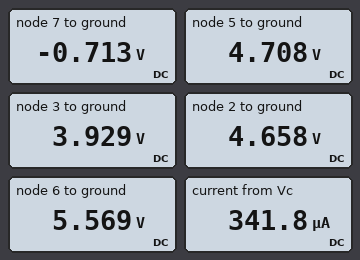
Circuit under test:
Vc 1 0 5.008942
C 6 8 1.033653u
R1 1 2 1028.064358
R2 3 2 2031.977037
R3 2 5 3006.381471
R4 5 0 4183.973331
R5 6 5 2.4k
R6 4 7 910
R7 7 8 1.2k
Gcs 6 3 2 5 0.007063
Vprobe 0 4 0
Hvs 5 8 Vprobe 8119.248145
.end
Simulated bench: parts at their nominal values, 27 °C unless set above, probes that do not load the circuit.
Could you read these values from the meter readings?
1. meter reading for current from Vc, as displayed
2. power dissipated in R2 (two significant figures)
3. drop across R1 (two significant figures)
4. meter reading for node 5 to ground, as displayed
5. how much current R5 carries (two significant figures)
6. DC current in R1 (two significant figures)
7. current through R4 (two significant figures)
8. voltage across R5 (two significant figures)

341.8 µA
260 µW
350 mV
4.708 V
360 µA
340 µA
1.1 mA
860 mV
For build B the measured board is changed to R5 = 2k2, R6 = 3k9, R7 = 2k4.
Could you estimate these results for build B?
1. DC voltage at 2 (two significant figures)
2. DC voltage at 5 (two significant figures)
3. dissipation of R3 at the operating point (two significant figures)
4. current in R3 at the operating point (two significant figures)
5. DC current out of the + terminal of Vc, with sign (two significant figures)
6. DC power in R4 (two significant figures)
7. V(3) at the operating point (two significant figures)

7.2 V
6.9 V
34 µW
110 µA
-2.1 mA
11 mW
12 V
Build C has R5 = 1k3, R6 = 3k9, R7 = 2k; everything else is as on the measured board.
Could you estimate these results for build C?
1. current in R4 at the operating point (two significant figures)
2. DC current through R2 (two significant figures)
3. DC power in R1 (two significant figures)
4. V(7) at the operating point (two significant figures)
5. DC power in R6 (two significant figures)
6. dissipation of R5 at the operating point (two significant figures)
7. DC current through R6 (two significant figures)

1.5 mA
1.4 mA
1.7 mW
-11 V
30 mW
2.4 mW
2.8 mA
